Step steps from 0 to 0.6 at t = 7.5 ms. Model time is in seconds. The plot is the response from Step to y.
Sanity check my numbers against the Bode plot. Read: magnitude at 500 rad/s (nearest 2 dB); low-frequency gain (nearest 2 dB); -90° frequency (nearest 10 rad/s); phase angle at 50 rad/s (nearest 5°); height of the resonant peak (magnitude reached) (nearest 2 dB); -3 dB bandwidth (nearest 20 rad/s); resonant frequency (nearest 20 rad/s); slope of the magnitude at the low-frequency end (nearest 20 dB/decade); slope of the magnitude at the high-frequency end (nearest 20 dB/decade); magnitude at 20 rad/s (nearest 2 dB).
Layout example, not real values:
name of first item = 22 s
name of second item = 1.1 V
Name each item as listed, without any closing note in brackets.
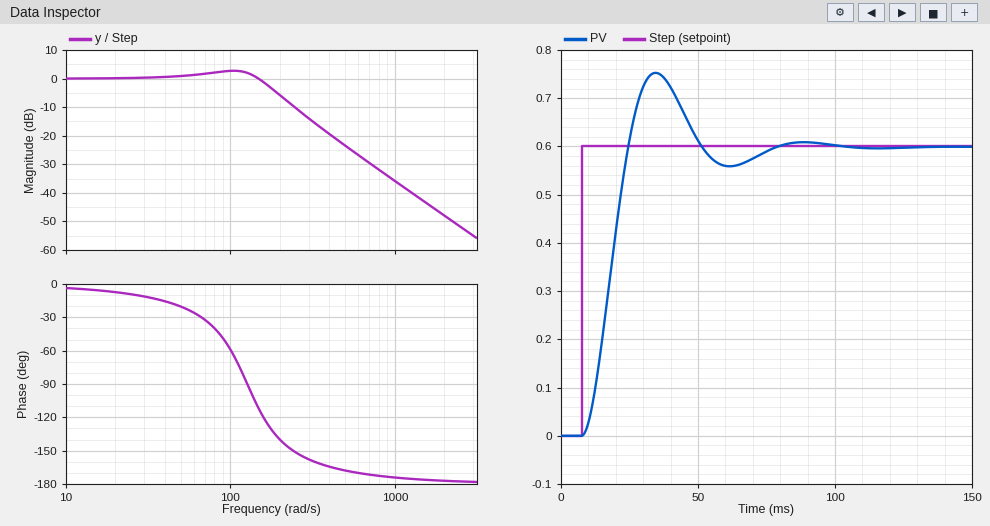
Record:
magnitude at 500 rad/s = -24 dB
low-frequency gain = 0 dB
-90° frequency = 130 rad/s
phase angle at 50 rad/s = -20°
height of the resonant peak (magnitude reached) = 2 dB
-3 dB bandwidth = 180 rad/s
resonant frequency = 100 rad/s
slope of the magnitude at the low-frequency end = 0 dB/decade
slope of the magnitude at the high-frequency end = -40 dB/decade
magnitude at 20 rad/s = 0 dB
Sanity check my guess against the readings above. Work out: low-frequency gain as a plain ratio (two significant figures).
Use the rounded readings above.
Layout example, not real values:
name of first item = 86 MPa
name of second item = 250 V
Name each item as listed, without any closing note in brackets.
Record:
low-frequency gain as a plain ratio = 1.0
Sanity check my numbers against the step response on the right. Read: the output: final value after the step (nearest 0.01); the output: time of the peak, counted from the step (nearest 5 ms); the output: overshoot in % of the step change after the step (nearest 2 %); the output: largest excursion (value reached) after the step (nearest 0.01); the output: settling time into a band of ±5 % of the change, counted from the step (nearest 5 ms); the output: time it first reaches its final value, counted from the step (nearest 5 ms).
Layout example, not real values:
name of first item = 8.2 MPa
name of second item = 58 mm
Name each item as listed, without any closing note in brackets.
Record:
the output: final value after the step = 0.60
the output: time of the peak, counted from the step = 25 ms
the output: overshoot in % of the step change after the step = 26 %
the output: largest excursion (value reached) after the step = 0.75
the output: settling time into a band of ±5 % of the change, counted from the step = 60 ms
the output: time it first reaches its final value, counted from the step = 15 ms
